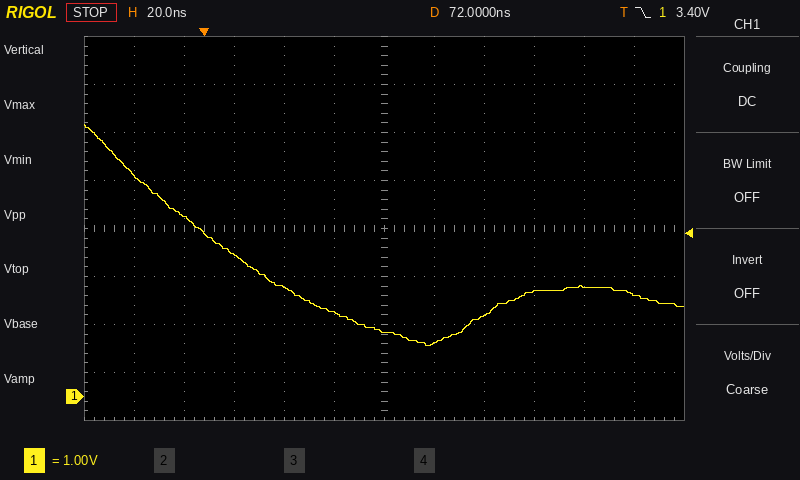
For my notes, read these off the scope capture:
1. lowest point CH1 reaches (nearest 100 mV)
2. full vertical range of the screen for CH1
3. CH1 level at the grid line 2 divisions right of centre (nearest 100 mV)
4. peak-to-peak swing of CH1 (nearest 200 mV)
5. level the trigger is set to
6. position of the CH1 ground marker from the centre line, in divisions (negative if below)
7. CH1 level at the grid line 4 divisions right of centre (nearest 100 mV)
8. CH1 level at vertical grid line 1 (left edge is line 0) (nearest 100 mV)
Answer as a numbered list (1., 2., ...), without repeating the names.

1. 1.1 V
2. 8 V
3. 1.7 V
4. 4.6 V
5. 3.40 V
6. -3.5 div
7. 2.3 V
8. 4.6 V
